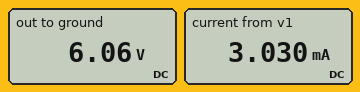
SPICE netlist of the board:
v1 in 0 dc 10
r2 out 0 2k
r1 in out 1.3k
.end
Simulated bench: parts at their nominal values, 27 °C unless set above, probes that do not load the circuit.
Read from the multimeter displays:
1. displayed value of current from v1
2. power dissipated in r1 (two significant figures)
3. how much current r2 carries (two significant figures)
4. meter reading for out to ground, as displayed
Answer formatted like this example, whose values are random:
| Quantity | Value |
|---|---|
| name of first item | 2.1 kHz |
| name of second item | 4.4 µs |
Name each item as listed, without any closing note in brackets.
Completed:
| Quantity | Value |
|---|---|
| displayed value of current from v1 | 3.030 mA |
| power dissipated in r1 | 12 mW |
| how much current r2 carries | 3.0 mA |
| meter reading for out to ground, as displayed | 6.06 V |
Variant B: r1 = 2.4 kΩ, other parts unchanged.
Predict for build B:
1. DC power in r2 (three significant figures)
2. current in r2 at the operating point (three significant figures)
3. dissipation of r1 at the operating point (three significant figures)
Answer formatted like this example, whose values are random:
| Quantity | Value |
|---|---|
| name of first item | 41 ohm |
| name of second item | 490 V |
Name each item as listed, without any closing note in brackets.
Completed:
| Quantity | Value |
|---|---|
| DC power in r2 | 10.3 mW |
| current in r2 at the operating point | 2.27 mA |
| dissipation of r1 at the operating point | 12.4 mW |
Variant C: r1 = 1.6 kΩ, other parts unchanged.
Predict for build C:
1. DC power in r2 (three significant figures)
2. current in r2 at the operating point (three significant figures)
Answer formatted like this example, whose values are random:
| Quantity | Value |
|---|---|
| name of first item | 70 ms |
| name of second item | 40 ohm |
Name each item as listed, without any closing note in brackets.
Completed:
| Quantity | Value |
|---|---|
| DC power in r2 | 15.4 mW |
| current in r2 at the operating point | 2.78 mA |
